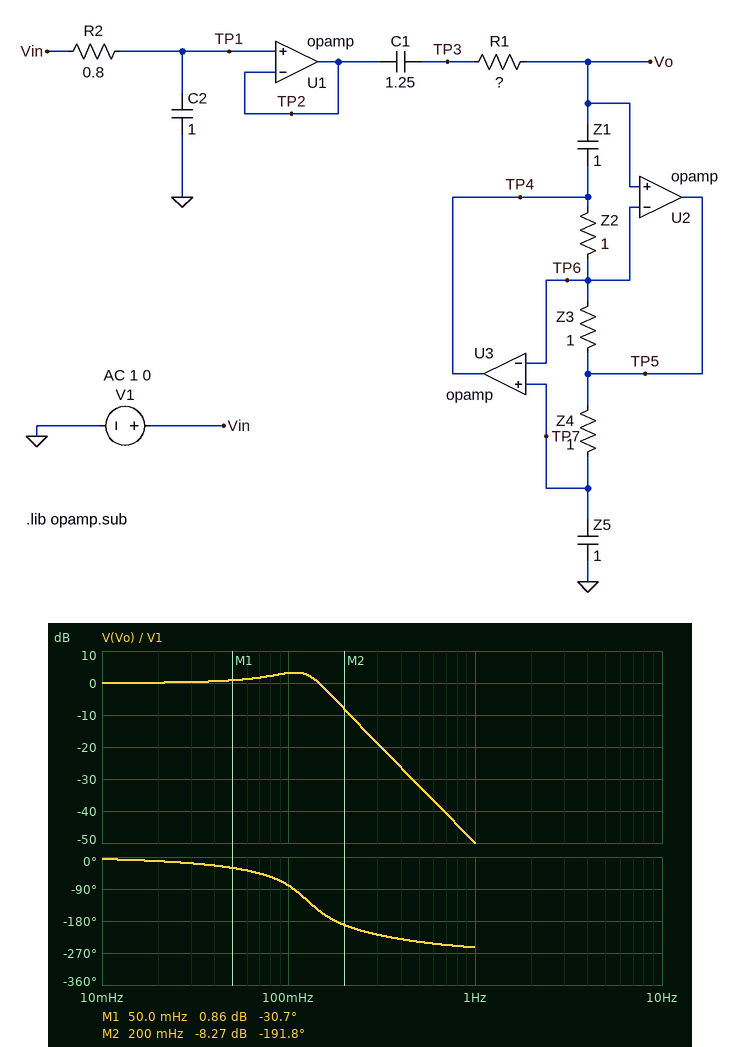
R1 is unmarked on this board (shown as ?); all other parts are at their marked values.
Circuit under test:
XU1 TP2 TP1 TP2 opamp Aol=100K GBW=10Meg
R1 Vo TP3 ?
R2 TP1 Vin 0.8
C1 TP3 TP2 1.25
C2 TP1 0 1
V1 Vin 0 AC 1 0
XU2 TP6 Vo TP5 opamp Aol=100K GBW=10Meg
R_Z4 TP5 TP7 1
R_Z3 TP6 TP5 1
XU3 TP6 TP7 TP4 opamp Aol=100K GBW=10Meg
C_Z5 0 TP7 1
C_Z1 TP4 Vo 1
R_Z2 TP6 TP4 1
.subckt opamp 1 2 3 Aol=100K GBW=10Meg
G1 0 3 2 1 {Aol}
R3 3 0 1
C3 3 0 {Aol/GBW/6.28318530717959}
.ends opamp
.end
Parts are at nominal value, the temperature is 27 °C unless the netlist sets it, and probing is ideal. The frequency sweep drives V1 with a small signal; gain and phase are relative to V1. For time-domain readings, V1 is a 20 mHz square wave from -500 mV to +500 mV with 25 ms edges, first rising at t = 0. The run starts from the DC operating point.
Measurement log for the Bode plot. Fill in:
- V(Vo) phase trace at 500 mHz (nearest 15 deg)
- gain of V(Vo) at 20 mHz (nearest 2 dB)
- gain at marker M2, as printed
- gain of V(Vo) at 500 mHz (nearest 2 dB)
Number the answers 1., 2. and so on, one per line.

1. -240 deg
2. 0 dB
3. -8.27 dB
4. -32 dB
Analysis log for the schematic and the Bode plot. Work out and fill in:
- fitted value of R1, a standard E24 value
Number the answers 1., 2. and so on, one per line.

1. 1.6 Ω
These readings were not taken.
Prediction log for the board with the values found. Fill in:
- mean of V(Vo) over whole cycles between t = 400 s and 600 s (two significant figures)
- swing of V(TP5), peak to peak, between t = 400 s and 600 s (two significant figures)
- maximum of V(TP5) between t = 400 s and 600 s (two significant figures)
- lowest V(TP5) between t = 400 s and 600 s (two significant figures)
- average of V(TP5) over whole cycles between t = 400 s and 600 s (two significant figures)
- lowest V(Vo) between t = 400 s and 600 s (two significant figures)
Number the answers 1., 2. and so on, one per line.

1. 500 mV
2. 1.8 V
3. 1.4 V
4. -390 mV
5. 500 mV
6. -280 mV
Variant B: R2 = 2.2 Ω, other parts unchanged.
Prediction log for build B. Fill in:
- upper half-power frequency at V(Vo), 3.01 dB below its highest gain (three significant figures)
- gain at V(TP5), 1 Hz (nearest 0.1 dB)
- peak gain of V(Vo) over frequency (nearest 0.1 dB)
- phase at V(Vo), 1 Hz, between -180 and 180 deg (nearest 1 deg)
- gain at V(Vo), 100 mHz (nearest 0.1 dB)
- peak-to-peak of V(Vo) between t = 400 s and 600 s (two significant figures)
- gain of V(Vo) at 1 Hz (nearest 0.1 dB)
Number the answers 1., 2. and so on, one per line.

1. 133 mHz
2. -42.7 dB
3. 0 dB
4. 99 deg
5. -0.5 dB
6. 1.1 V
7. -58.7 dB
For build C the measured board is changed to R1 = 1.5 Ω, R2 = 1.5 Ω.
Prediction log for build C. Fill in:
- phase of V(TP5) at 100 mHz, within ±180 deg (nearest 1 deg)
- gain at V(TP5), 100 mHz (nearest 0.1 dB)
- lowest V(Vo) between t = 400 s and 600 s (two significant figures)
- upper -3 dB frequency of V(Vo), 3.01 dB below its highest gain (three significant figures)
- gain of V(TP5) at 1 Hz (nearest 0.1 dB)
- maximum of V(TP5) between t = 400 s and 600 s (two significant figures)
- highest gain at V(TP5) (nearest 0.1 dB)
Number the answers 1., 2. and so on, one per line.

1. -62 deg
2. 2.5 dB
3. -160 mV
4. 143 mHz
5. -38.8 dB
6. 1.2 V
7. 2.7 dB
